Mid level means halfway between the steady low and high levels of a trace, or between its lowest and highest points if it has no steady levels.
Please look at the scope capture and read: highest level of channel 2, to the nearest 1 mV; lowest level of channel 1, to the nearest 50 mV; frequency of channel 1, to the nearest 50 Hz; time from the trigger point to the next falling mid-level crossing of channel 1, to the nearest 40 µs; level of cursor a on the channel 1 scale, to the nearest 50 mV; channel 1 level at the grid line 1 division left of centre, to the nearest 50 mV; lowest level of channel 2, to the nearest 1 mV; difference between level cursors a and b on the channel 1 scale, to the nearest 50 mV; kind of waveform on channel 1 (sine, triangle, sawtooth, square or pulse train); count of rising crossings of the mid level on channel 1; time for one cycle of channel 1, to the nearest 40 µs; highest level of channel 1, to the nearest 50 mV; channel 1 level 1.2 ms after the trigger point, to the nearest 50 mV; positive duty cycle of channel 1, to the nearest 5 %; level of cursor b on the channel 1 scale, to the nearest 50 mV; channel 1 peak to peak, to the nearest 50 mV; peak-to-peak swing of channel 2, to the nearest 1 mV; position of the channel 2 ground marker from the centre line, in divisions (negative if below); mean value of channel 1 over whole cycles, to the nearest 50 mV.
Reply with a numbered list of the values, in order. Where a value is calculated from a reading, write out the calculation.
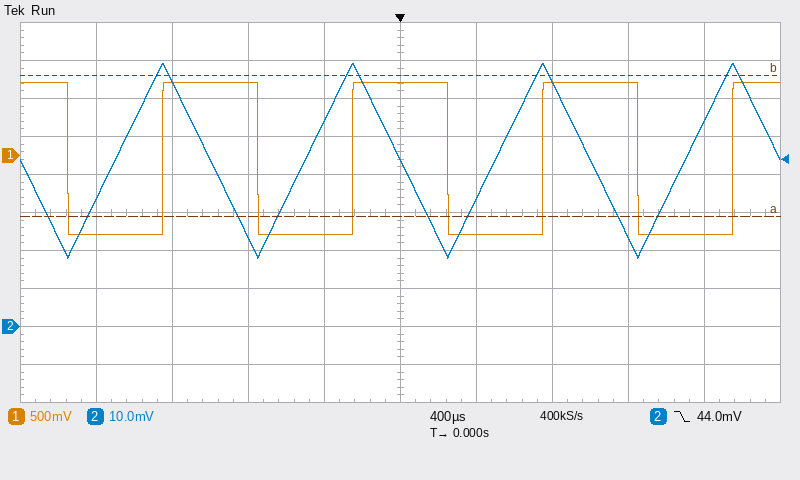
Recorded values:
1. 69 mV
2. -1.05 V
3. 1 / 1.00 ms ≈ 1.00 kHz
4. 240 µs
5. -800 mV
6. -1.05 V
7. 18 mV
8. 1.85 V
9. square
10. 4
11. 1.00 ms
12. 950 mV
13. 950 mV
14. 50 %
15. 1.05 V
16. 950 mV − (-1.05 V) = 2.00 V
17. 69 mV − (18 mV) = 51 mV
18. -3.0 div
19. -1.05 V + 0.5 × (950 mV − (-1.05 V)) ≈ -50 mV
